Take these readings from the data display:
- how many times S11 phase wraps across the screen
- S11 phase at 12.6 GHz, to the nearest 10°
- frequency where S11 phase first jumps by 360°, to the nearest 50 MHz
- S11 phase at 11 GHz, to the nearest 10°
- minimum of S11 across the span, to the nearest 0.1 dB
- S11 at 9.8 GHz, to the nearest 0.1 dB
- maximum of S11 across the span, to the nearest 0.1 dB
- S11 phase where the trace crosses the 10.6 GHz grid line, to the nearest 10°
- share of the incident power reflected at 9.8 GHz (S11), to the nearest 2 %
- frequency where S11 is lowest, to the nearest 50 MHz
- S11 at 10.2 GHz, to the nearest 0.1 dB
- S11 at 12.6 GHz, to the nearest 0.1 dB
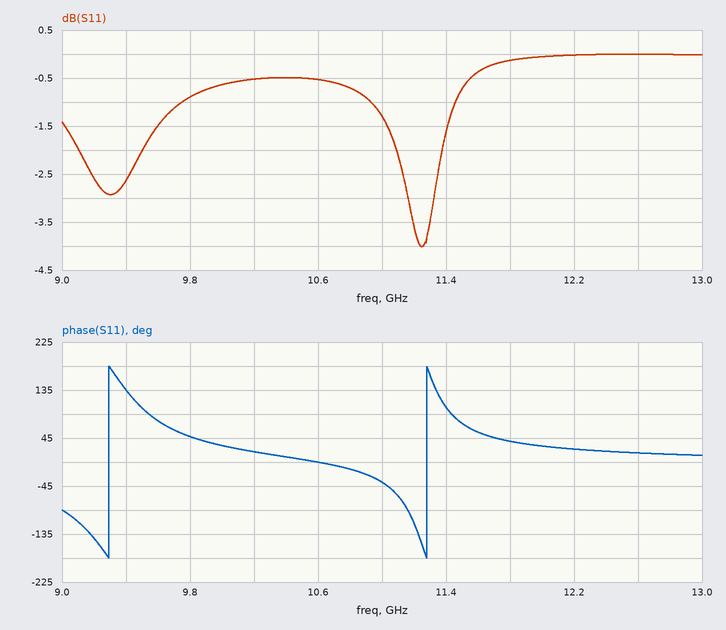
2
20°
9.30 GHz
-40°
-4.0 dB
-0.9 dB
0.0 dB
0°
82 %
11.25 GHz
-0.5 dB
0.0 dB
